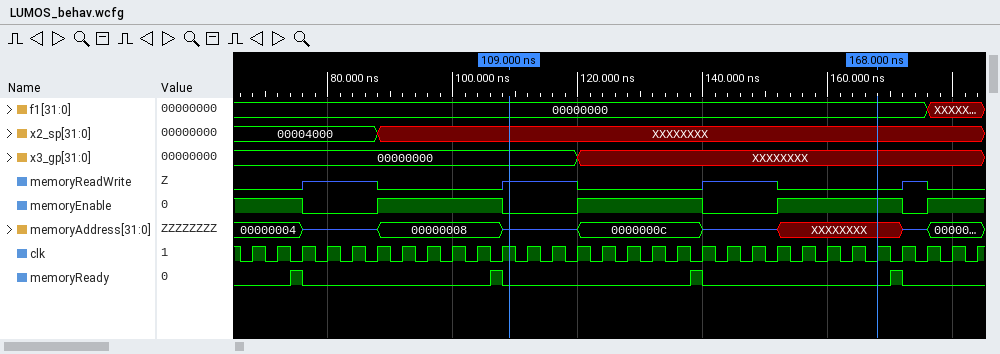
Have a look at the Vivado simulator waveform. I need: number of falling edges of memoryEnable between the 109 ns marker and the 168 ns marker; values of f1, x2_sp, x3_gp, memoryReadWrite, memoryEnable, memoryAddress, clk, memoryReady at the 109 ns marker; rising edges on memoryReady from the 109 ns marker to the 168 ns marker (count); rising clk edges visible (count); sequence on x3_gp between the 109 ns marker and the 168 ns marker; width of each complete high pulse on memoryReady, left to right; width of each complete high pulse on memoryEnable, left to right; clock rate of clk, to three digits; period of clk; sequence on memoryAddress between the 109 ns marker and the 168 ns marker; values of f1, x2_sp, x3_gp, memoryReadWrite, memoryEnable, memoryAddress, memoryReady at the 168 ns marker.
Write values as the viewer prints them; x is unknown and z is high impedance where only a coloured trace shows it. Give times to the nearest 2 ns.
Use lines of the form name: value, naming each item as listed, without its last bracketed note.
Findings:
number of falling edges of memoryEnable between the 109 ns marker and the 168 ns marker: 1
values of f1, x2_sp, x3_gp, memoryReadWrite, memoryEnable, memoryAddress, clk, memoryReady at the 109 ns marker: f1=00000000, x2_sp=XXXXXXXX, x3_gp=00000000, memoryReadWrite=z, memoryEnable=0, memoryAddress=z, clk=1, memoryReady=0
rising edges on memoryReady from the 109 ns marker to the 168 ns marker: 1
rising clk edges visible: 30
sequence on x3_gp between the 109 ns marker and the 168 ns marker: 00000000, XXXXXXXX
width of each complete high pulse on memoryReady, left to right: 2 ns, 2 ns, 2 ns, 2 ns
width of each complete high pulse on memoryEnable, left to right: 20 ns, 20 ns, 20 ns
clock rate of clk, to three digits: 250 MHz
period of clk: 4 ns
sequence on memoryAddress between the 109 ns marker and the 168 ns marker: z, 0000000c, z, XXXXXXXX
values of f1, x2_sp, x3_gp, memoryReadWrite, memoryEnable, memoryAddress, memoryReady at the 168 ns marker: f1=00000000, x2_sp=XXXXXXXX, x3_gp=XXXXXXXX, memoryReadWrite=0, memoryEnable=1, memoryAddress=XXXXXXXX, memoryReady=0
